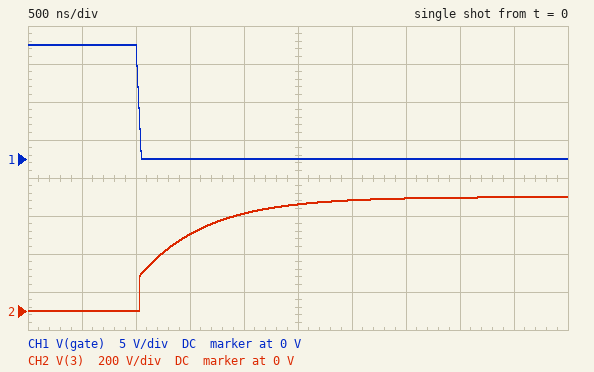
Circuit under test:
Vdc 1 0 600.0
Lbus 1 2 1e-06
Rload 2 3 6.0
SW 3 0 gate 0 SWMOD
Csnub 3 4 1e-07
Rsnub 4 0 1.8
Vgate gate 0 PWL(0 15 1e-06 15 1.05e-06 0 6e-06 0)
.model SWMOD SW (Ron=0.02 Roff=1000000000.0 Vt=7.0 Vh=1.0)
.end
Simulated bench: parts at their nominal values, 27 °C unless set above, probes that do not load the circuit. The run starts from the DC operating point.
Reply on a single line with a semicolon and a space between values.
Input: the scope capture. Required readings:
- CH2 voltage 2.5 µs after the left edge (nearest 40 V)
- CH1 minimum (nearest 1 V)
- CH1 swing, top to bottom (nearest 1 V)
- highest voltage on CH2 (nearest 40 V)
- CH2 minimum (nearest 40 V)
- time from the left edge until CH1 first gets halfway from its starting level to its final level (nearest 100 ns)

560 V; 0 V; 15 V; 600 V; 0 V; 1.0 µs
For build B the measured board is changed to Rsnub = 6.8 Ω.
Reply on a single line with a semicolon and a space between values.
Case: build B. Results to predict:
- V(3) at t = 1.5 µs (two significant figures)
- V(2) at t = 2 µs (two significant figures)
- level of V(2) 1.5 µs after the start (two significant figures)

440 V; 620 V; 630 V
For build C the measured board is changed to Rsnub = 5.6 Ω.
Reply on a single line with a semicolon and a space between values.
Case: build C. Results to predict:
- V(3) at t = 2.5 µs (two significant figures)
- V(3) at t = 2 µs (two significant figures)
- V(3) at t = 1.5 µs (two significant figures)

530 V; 490 V; 430 V
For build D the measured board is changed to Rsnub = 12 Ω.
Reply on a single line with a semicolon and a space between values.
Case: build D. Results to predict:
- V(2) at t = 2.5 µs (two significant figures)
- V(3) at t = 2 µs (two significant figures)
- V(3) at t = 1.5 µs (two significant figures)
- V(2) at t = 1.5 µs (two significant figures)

610 V; 500 V; 470 V; 610 V
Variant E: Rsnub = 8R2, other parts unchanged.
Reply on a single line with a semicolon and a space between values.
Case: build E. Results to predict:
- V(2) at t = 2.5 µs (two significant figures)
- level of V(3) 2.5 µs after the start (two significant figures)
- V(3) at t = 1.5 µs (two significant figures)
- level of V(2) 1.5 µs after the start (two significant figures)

610 V; 530 V; 450 V; 620 V
